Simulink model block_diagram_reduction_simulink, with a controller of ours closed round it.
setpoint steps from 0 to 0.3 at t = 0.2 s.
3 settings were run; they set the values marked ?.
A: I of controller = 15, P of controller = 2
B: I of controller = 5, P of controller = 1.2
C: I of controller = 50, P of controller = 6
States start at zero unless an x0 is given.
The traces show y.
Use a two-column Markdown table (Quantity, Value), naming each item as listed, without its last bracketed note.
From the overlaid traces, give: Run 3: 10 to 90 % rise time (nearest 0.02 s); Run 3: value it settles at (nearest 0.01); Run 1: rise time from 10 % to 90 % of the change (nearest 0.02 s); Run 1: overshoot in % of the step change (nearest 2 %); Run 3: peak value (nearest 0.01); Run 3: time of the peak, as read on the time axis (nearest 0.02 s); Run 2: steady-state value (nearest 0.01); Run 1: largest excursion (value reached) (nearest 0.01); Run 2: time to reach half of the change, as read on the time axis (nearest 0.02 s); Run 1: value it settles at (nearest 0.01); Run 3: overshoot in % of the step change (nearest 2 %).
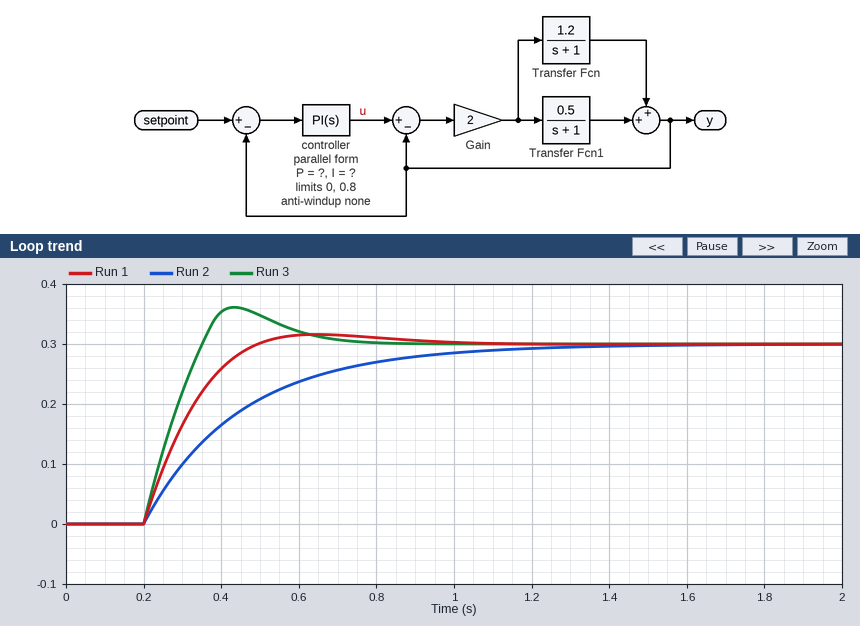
| Quantity | Value |
|---|---|
| Run 3: 10 to 90 % rise time | 0.12 s |
| Run 3: value it settles at | 0.30 |
| Run 1: rise time from 10 % to 90 % of the change | 0.20 s |
| Run 1: overshoot in % of the step change | 6 % |
| Run 3: peak value | 0.36 |
| Run 3: time of the peak, as read on the time axis | 0.44 s |
| Run 2: steady-state value | 0.30 |
| Run 1: largest excursion (value reached) | 0.32 |
| Run 2: time to reach half of the change, as read on the time axis | 0.38 s |
| Run 1: value it settles at | 0.30 |
| Run 3: overshoot in % of the step change | 20 % |
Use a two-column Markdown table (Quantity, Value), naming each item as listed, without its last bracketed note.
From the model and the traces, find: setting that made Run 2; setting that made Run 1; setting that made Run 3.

| Quantity | Value |
|---|---|
| setting that made Run 2 | B |
| setting that made Run 1 | A |
| setting that made Run 3 | C |
